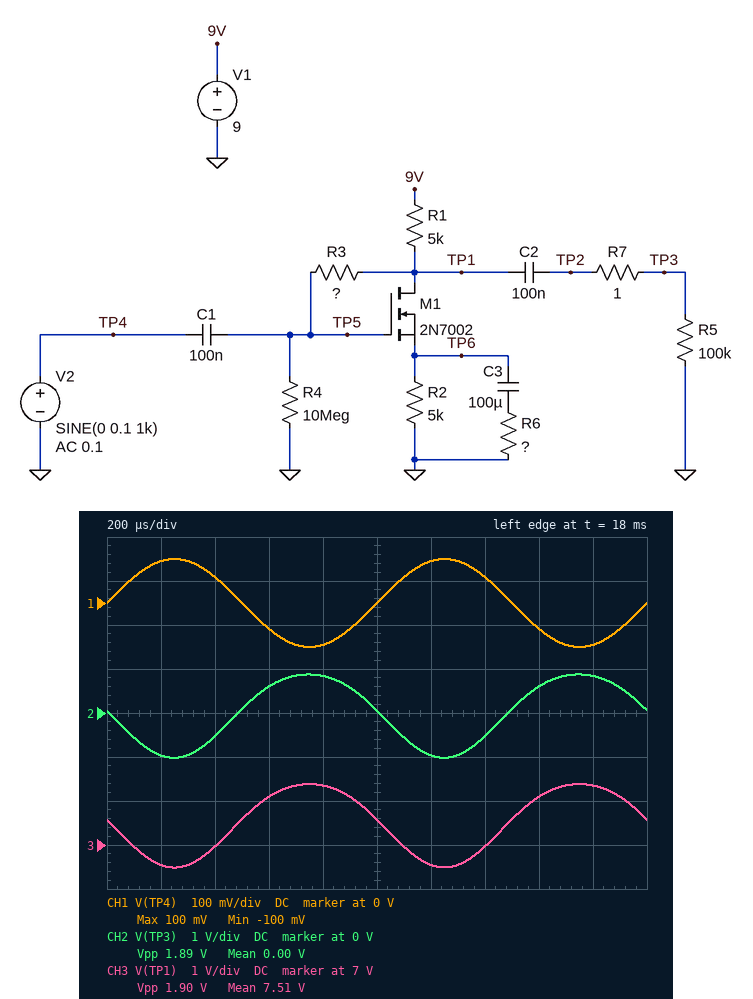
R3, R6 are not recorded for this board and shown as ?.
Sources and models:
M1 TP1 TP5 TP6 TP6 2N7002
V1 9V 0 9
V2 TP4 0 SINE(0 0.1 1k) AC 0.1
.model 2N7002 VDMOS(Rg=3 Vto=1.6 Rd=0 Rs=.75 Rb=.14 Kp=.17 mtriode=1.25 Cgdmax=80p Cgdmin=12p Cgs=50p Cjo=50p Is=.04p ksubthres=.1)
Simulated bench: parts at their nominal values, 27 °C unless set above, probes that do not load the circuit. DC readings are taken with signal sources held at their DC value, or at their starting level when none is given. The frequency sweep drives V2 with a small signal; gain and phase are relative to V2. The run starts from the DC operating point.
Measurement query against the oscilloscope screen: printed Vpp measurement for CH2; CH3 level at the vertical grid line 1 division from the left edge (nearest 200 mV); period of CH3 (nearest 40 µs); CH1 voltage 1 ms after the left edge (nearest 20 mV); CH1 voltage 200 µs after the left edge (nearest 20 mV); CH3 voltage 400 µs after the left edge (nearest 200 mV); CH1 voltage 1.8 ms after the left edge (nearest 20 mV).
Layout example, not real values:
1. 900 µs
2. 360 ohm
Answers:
1. 1.89 V
2. 6.6 V
3. 1.00 ms
4. 0 V
5. 100 mV
6. 7.0 V
7. -100 mV
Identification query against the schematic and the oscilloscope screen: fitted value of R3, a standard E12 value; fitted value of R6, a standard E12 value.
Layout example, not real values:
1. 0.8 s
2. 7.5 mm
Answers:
1. 15 MΩ
2. 270 Ω
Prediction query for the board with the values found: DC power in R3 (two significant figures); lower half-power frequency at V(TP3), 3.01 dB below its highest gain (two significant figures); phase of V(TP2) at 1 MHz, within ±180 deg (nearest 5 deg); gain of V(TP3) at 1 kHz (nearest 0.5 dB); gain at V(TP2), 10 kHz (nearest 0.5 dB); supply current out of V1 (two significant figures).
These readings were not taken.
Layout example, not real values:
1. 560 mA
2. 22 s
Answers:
1. 1.4 µW
2. 16 Hz
3. 135 deg
4. 20.0 dB
5. 20.0 dB
6. 290 µA
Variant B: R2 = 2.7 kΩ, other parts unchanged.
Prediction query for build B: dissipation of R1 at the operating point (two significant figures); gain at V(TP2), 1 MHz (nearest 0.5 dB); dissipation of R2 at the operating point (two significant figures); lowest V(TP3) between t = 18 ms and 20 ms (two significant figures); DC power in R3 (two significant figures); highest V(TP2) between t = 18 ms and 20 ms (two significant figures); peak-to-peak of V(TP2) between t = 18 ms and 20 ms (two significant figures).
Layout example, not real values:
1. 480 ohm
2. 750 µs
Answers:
1. 900 µW
2. 19.5 dB
3. 490 µW
4. -1.2 V
5. 1.1 µW
6. 1.1 V
7. 2.3 V
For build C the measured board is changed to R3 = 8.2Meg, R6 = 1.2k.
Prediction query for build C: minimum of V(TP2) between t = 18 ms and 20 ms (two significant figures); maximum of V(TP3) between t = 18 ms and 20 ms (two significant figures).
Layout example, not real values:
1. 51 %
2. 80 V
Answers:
1. -420 mV
2. 420 mV
